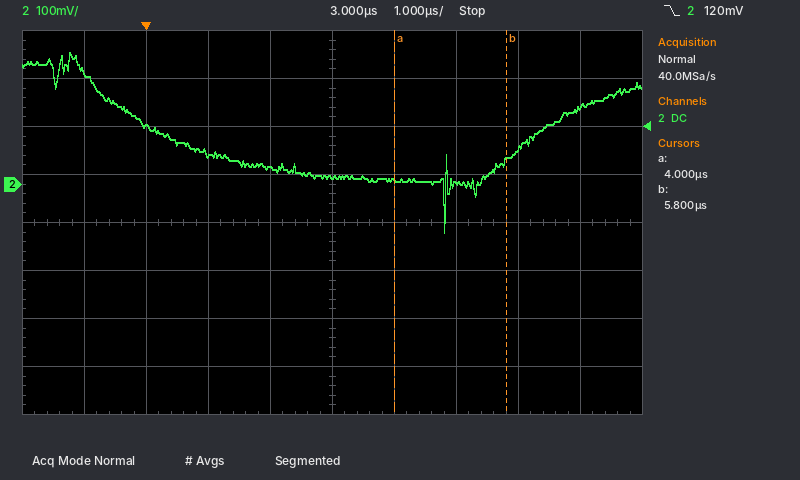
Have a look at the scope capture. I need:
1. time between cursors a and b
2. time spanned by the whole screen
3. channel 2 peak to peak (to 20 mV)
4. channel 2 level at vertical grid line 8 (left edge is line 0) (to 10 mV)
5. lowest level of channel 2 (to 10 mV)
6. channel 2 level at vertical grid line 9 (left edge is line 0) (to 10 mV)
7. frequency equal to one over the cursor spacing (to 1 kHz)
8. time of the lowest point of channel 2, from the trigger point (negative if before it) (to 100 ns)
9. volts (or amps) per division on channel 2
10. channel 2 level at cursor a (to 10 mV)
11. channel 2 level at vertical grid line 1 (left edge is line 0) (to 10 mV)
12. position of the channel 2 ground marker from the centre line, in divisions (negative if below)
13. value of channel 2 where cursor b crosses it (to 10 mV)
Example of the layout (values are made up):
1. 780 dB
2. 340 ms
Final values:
1. 1.8 µs
2. 10 µs
3. 380 mV
4. 70 mV
5. -100 mV
6. 160 mV
7. 556 kHz
8. +4.8 µs
9. 100 mV
10. 10 mV
11. 230 mV
12. +0.8 div
13. 50 mV
